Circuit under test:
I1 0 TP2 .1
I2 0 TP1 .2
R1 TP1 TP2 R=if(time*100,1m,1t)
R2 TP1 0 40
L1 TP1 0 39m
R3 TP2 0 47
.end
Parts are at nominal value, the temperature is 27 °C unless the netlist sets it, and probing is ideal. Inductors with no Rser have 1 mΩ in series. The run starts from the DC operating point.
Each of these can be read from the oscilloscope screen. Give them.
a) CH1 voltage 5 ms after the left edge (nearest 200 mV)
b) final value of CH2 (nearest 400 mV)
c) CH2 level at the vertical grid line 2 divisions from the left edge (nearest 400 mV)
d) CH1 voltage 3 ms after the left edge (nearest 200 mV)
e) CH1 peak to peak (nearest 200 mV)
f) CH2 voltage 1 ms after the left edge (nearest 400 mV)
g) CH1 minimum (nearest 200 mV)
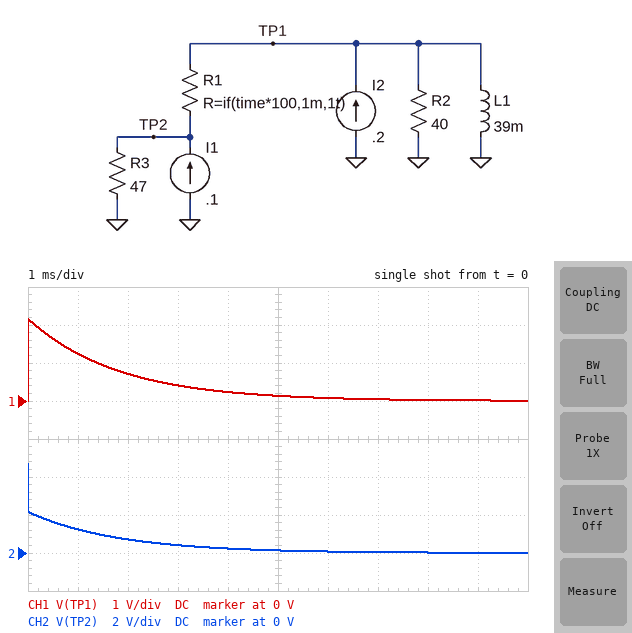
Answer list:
200 mV
0 V
800 mV
400 mV
2.2 V
1.2 V
0 V
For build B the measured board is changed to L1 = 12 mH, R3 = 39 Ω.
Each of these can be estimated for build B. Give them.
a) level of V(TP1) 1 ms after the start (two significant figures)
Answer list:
380 mV
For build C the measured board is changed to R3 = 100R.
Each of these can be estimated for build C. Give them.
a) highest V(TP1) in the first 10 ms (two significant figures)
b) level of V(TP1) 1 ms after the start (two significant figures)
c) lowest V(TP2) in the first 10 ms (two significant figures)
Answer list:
2.9 V
1.4 V
2.3 mV
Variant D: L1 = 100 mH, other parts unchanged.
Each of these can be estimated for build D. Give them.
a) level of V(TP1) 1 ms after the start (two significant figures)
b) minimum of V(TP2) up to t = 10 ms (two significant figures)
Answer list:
1.7 V
250 mV
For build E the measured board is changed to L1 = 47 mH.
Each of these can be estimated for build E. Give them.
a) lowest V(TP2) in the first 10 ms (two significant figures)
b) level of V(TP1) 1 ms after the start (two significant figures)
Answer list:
22 mV
1.4 V
